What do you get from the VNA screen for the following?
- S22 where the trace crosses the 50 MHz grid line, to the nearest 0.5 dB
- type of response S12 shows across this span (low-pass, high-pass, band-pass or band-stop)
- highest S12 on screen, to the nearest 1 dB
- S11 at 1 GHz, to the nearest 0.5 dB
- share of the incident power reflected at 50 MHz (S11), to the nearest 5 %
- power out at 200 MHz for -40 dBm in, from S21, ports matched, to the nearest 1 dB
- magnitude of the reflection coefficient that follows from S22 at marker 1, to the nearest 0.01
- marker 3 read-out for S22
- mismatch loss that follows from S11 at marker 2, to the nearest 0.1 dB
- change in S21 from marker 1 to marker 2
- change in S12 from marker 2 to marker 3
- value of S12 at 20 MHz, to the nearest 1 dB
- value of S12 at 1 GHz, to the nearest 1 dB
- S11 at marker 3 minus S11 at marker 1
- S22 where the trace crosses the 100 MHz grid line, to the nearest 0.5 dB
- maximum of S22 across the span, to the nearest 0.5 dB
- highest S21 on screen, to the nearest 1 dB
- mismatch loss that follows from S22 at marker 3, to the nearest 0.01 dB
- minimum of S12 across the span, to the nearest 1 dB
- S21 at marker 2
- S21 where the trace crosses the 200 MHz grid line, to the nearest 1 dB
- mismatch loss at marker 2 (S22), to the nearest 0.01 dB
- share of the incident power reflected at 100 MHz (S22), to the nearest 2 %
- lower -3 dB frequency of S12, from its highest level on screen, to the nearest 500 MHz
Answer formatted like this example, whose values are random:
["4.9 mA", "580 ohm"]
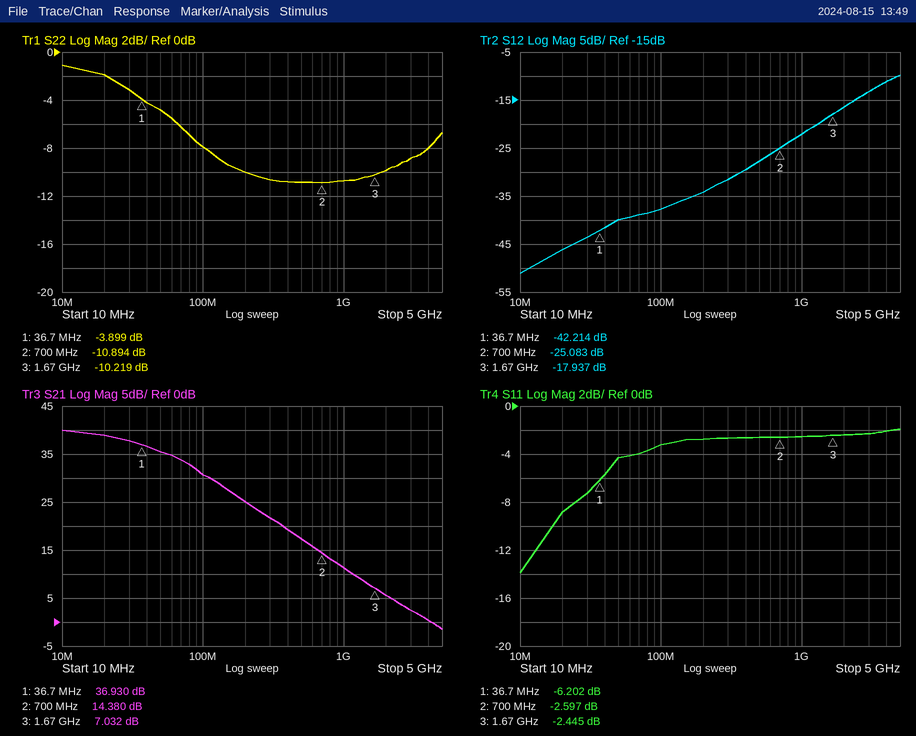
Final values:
["-5.0 dB", "high-pass", "-10 dB", "-2.5 dB", "35 %", "-15 dBm", "0.64", "-10.219 dB", "3.5 dB", "-22.550 dB", "7.146 dB", "-46 dB", "-22 dB", "3.757 dB", "-8.0 dB", "-1.0 dB", "40 dB", "0.43 dB", "-51 dB", "14.380 dB", "25 dB", "0.37 dB", "16 %", "3.0 GHz"]
